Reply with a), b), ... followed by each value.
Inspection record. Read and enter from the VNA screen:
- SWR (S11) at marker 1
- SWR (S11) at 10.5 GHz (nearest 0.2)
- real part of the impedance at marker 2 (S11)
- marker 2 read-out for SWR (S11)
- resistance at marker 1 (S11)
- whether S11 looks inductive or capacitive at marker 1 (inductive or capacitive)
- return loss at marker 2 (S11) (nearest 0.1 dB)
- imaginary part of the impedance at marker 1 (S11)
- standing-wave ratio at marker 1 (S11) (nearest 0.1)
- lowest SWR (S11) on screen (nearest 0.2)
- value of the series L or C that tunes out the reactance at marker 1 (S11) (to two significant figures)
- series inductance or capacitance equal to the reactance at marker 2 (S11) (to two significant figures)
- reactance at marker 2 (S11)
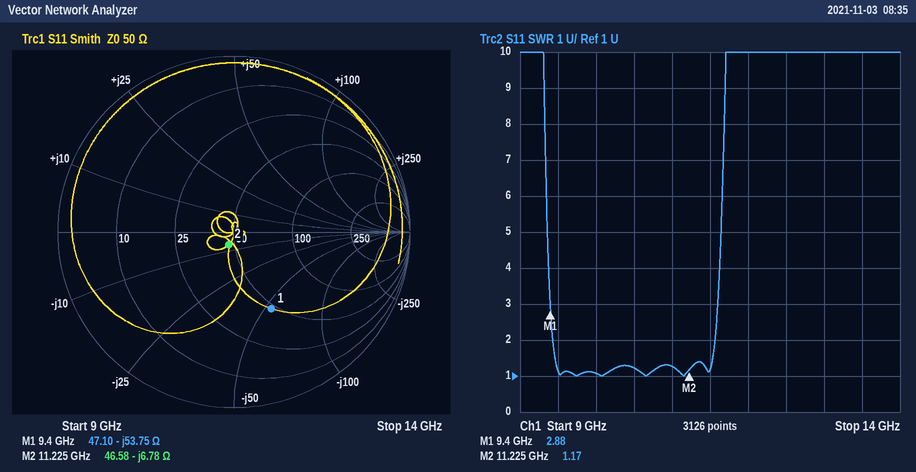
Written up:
a) 2.88
b) 1.2
c) 46.58 Ω
d) 1.17
e) 47.10 Ω
f) capacitive
g) 22.1 dB
h) -53.75 Ω
i) 2.9
j) 1.0
k) 910 pH
l) 2.1 pF
m) -6.78 Ω
